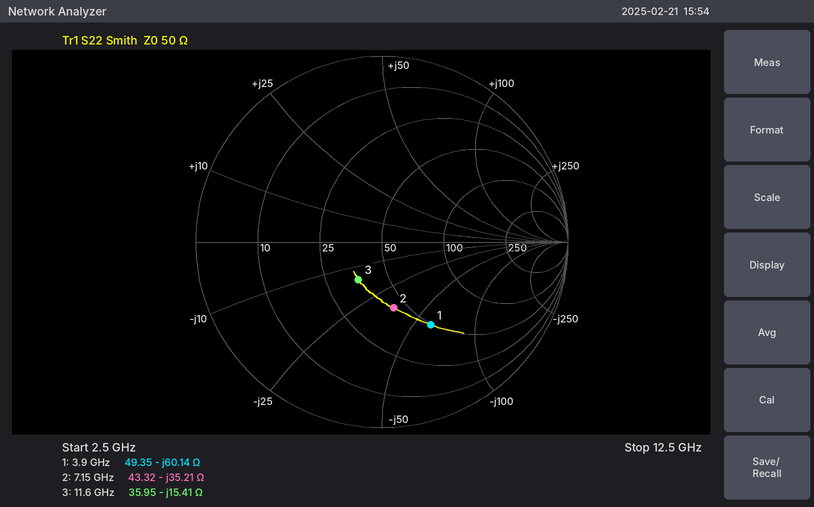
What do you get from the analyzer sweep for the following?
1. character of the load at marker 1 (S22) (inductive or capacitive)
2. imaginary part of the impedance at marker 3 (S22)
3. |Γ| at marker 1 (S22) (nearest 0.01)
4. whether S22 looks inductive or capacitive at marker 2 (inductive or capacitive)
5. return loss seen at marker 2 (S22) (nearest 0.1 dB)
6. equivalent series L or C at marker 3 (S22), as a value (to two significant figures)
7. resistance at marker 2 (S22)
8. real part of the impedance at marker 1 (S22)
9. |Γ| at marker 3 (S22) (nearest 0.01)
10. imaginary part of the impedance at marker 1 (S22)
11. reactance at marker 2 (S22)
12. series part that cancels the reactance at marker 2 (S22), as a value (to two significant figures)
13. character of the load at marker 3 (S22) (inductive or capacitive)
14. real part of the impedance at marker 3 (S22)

capacitive
-15.41 Ω
0.52
capacitive
8.9 dB
890 fF
43.32 Ω
49.35 Ω
0.24
-60.14 Ω
-35.21 Ω
780 pH
capacitive
35.95 Ω
